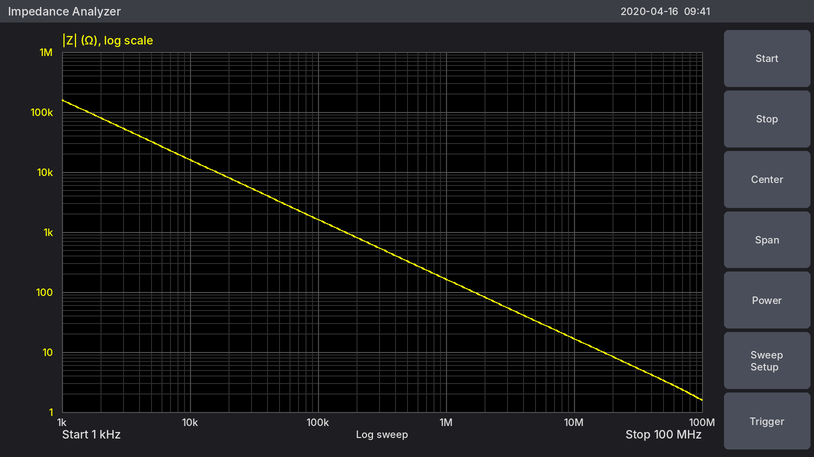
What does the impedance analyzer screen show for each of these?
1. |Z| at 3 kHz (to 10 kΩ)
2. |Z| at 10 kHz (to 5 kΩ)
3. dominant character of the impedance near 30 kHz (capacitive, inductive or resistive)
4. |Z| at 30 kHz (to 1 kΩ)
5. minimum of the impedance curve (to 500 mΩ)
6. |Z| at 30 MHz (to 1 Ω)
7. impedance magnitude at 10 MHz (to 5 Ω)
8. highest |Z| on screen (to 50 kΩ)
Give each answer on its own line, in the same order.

50 kΩ
15 kΩ
capacitive
5 kΩ
1.5 Ω
6 Ω
15 Ω
150 kΩ
